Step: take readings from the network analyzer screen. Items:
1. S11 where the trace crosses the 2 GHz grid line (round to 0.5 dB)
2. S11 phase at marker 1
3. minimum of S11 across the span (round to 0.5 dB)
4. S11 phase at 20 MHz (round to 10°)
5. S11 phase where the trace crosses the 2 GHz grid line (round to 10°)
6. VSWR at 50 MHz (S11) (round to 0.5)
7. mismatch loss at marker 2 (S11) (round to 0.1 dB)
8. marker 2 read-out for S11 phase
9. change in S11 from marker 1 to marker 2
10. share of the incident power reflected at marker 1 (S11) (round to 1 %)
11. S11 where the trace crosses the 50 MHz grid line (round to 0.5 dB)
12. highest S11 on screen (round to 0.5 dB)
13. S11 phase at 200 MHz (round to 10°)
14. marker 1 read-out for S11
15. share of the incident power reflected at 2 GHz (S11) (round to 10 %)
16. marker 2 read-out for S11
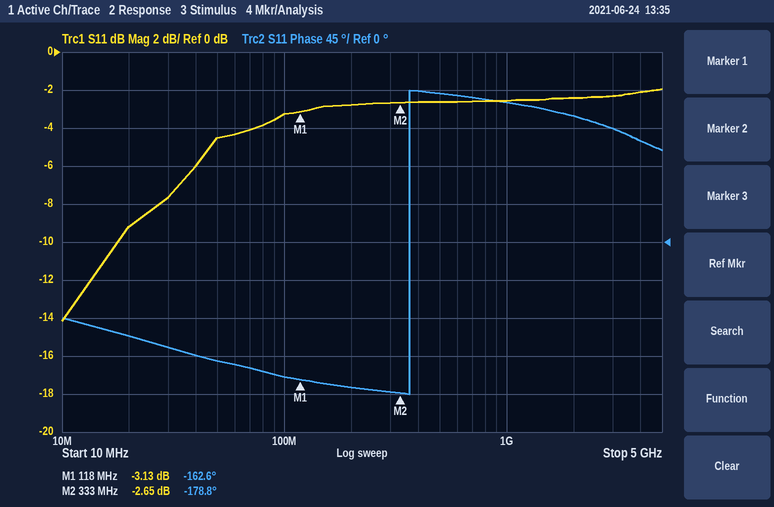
-2.5 dB
-162.6°
-14.0 dB
-110°
150°
4.0
3.4 dB
-178.8°
0.48 dB
49 %
-4.5 dB
-2.0 dB
-170°
-3.13 dB
60 %
-2.65 dB
